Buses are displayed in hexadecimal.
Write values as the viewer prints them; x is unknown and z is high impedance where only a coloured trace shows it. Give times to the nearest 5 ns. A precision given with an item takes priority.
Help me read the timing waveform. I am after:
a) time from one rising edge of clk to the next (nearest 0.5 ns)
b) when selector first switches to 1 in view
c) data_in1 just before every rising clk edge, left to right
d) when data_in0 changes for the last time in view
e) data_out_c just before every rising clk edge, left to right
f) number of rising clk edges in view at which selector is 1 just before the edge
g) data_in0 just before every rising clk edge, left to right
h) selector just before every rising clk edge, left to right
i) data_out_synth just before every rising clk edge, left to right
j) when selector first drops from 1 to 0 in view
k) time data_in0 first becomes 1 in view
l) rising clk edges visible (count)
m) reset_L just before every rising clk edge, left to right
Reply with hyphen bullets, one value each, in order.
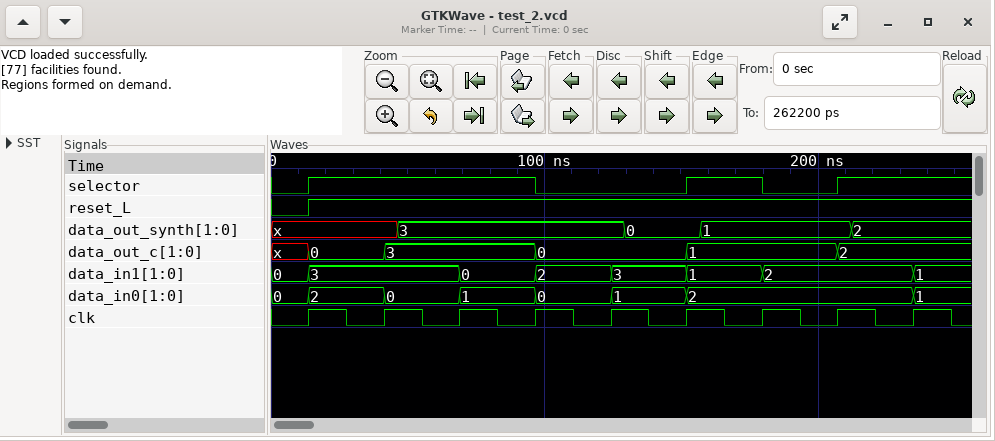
- 27.5 ns
- 15 ns
- 0, 3, 3, 0, 2, 3, 1, 2, 2
- 235 ns
- x, 0, 3, 3, 0, 0, 1, 1, 2
- 5
- 0, 2, 0, 1, 0, 1, 2, 2, 2
- 0 1 1 1 0 0 1 0 1
- x, x, 3, 3, 3, 0, 1, 1, 2
- 95 ns
- 70 ns
- 9
- 0 1 1 1 1 1 1 1 1
